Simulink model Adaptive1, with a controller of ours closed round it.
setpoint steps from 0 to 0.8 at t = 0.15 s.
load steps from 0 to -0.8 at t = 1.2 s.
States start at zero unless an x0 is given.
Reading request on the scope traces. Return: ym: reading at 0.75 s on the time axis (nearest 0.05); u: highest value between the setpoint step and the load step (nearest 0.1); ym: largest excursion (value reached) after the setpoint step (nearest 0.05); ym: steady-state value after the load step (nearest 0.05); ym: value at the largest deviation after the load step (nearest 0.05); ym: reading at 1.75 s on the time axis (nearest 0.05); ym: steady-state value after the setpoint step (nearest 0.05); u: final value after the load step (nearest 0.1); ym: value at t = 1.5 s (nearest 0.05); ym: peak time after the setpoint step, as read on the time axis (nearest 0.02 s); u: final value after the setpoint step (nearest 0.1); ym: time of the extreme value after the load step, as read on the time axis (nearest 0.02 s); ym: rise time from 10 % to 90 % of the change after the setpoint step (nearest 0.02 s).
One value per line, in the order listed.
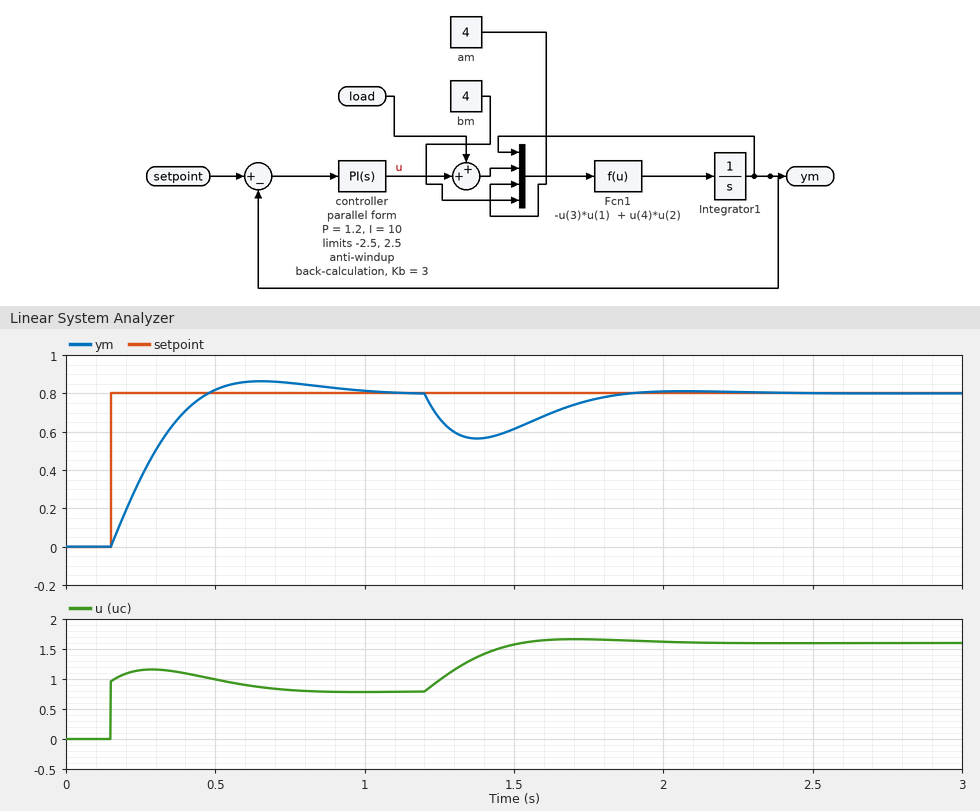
0.85
1.2
0.85
0.80
0.55
0.75
0.80
1.6
0.60
0.66 s
0.8
1.38 s
0.24 s
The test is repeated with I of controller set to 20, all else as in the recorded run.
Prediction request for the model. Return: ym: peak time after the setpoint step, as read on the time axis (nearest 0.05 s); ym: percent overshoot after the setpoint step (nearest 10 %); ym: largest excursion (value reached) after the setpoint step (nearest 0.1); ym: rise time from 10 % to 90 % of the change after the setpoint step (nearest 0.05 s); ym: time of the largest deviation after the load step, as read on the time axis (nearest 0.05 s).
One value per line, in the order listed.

0.50 s
20 %
1.0
0.15 s
1.35 s
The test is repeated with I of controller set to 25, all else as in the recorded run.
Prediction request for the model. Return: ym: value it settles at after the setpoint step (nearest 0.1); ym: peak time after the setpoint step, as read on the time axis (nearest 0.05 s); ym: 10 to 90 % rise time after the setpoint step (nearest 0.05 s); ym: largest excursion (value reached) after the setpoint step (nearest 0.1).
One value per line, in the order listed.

0.8
0.45 s
0.15 s
1.0
